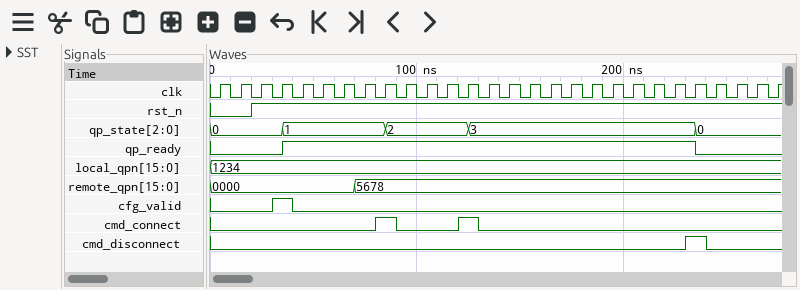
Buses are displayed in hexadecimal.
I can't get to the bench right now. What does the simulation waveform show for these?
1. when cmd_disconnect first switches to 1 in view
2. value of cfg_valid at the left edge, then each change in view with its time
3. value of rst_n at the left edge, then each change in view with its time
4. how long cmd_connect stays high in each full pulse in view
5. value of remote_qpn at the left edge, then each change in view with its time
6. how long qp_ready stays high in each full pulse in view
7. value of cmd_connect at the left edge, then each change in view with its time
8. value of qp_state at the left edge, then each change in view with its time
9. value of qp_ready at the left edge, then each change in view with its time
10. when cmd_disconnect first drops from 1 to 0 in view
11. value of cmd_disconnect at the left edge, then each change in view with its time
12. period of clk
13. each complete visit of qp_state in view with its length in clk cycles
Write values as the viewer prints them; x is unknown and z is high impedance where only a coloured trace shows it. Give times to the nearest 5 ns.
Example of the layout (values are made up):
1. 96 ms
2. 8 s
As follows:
1. 230 ns
2. 0, 1 at 30 ns, 0 at 40 ns
3. 0, 1 at 20 ns
4. 10 ns, 10 ns
5. 0000, 5678 at 70 ns
6. 200 ns
7. 0, 1 at 80 ns, 0 at 90 ns, 1 at 120 ns, 0 at 130 ns
8. 0, 1 at 35 ns, 2 at 85 ns, 3 at 125 ns, 0 at 235 ns
9. 0, 1 at 35 ns, 0 at 235 ns
10. 240 ns
11. 0, 1 at 230 ns, 0 at 240 ns
12. 10 ns
13. 1: 5, 2: 4, 3: 11
